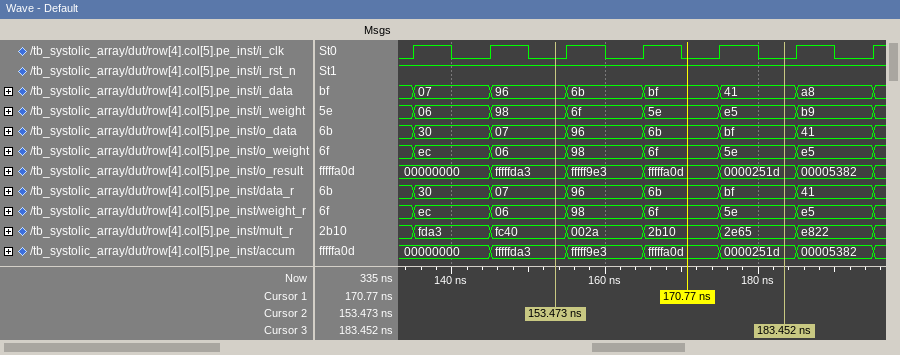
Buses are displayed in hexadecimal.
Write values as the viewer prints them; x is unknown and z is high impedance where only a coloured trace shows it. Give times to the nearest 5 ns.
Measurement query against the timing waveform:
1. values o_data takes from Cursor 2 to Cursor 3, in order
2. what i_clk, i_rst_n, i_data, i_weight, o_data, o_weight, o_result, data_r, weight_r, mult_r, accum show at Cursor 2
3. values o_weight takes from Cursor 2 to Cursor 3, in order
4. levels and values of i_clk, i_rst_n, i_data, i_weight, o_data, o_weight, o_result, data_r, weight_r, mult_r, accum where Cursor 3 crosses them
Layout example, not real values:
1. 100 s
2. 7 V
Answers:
1. 07, 96, 6b, bf
2. i_clk=0, i_rst_n=1, i_data=96, i_weight=98, o_data=07, o_weight=06, o_result=fffffda3, data_r=07, weight_r=06, mult_r=fc40, accum=fffffda3
3. 06, 98, 6f, 5e
4. i_clk=0, i_rst_n=1, i_data=41, i_weight=e5, o_data=bf, o_weight=5e, o_result=0000251d, data_r=bf, weight_r=5e, mult_r=2e65, accum=0000251d
